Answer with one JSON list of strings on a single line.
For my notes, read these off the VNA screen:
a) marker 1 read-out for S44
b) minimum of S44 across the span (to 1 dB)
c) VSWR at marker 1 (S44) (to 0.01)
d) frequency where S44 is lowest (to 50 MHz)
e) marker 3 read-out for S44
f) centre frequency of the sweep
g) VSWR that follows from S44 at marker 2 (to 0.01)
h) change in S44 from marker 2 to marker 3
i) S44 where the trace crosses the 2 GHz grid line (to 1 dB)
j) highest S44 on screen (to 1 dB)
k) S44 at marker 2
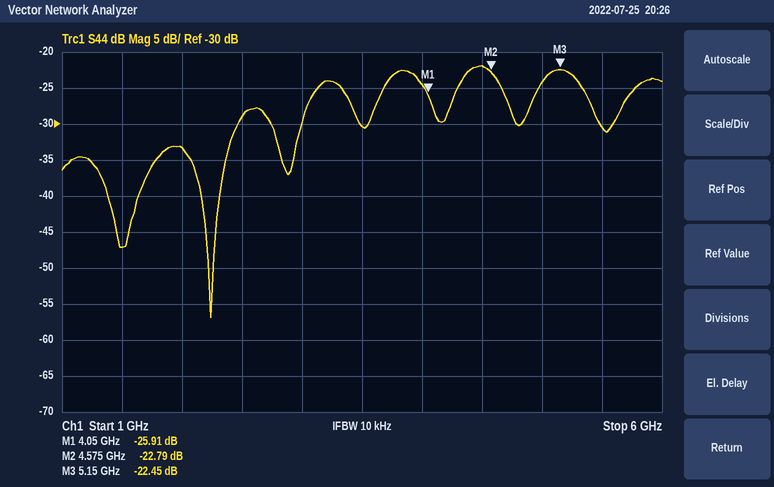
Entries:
["-25.91 dB", "-57 dB", "1.11", "2.25 GHz", "-22.45 dB", "3.5 GHz", "1.16", "0.34 dB", "-33 dB", "-22 dB", "-22.79 dB"]
